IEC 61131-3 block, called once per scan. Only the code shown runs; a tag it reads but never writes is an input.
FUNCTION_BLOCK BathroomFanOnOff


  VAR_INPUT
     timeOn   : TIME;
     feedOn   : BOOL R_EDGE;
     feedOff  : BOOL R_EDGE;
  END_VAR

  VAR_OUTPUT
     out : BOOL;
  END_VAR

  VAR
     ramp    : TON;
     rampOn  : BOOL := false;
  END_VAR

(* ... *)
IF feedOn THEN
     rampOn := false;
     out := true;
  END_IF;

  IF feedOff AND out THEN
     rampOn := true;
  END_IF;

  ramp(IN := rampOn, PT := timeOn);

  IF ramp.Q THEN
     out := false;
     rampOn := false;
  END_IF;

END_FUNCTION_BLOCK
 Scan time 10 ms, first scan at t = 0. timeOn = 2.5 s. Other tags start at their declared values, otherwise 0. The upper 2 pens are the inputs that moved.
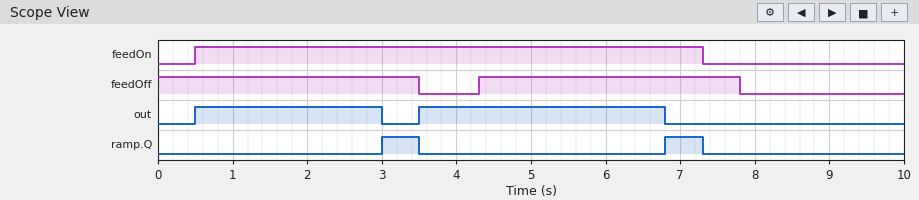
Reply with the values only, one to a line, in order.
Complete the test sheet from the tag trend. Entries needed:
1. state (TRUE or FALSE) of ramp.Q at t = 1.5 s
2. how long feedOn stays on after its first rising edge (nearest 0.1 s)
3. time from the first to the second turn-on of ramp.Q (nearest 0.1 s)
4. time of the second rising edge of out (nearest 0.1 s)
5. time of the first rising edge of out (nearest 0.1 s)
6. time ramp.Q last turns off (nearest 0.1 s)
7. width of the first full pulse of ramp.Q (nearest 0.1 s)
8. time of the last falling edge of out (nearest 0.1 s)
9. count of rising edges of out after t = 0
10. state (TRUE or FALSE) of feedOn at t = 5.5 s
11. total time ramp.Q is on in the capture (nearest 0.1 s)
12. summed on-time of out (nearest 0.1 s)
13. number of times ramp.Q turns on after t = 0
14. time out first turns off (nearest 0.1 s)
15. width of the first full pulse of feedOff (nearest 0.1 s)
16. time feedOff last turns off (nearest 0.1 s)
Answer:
FALSE
6.8 s
3.8 s
3.5 s
0.5 s
7.3 s
0.5 s
6.8 s
2
TRUE
1.0 s
5.8 s
2
3.0 s
3.5 s
7.8 s
